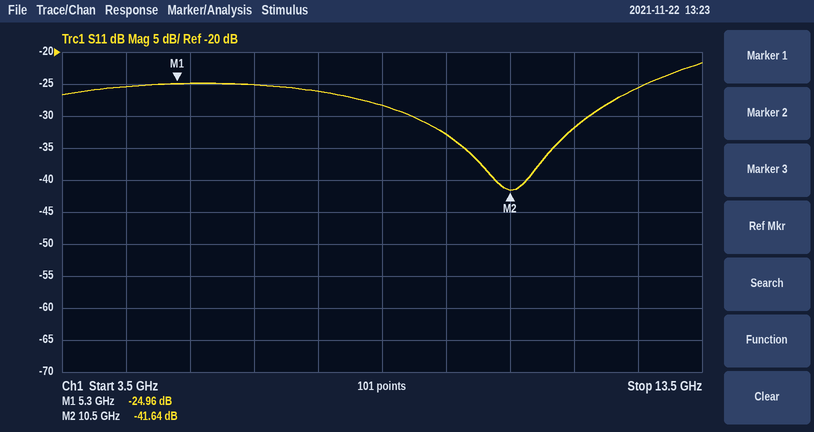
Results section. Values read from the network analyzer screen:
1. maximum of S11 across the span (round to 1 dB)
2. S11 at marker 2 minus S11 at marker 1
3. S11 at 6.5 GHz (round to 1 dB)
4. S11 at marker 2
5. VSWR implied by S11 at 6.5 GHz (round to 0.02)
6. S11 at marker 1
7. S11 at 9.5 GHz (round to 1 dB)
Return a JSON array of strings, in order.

["-22 dB", "-16.68 dB", "-25 dB", "-41.64 dB", "1.12", "-24.96 dB", "-33 dB"]
